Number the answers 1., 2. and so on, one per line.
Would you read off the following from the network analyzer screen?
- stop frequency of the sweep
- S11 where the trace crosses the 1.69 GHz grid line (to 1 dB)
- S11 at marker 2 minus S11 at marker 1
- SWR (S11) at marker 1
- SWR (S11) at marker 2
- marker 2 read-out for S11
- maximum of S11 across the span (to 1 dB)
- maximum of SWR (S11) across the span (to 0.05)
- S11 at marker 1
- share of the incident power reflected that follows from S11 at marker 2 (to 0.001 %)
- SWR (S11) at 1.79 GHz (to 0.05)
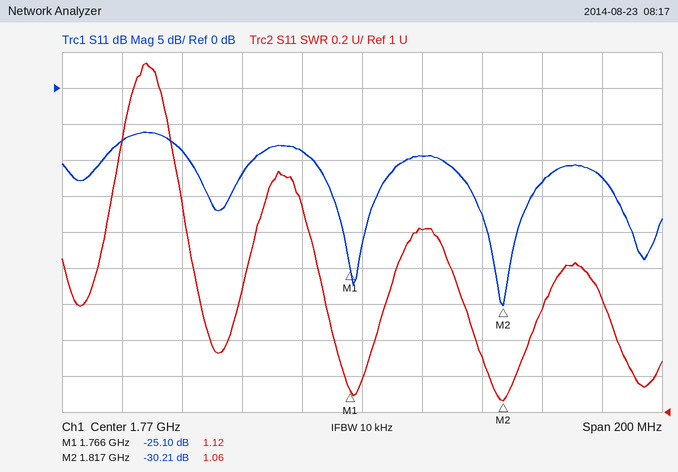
1. 1.87 GHz
2. -7 dB
3. -5.11 dB
4. 1.12
5. 1.06
6. -30.21 dB
7. -6 dB
8. 2.95
9. -25.10 dB
10. 0.095 %
11. 2.00
